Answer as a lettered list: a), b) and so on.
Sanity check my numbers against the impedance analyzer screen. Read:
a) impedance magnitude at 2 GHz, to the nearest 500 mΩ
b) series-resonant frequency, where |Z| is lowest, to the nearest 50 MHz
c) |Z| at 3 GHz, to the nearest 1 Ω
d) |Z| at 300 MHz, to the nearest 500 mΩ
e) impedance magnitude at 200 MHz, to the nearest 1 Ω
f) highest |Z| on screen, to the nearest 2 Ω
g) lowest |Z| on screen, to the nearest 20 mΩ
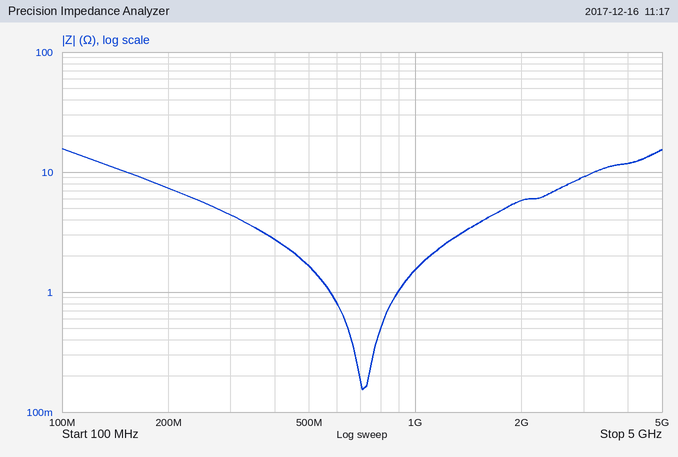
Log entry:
a) 6.0 Ω
b) 700 MHz
c) 9 Ω
d) 4.5 Ω
e) 7 Ω
f) 16 Ω
g) 160 mΩ
